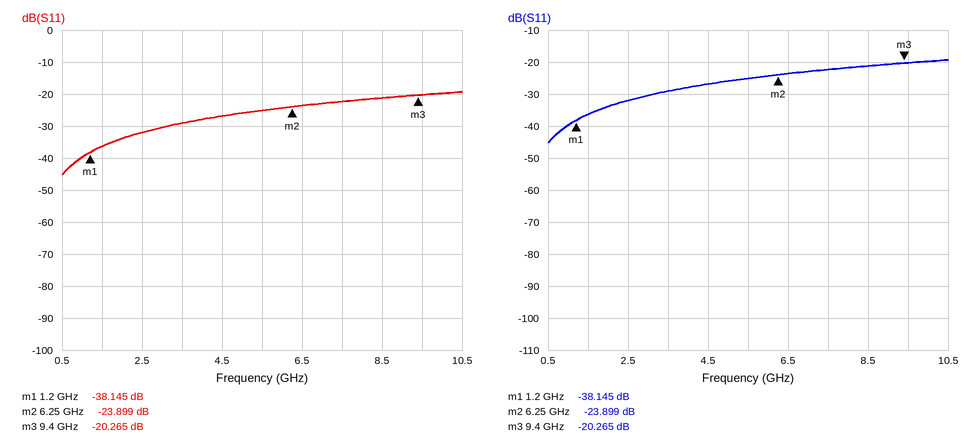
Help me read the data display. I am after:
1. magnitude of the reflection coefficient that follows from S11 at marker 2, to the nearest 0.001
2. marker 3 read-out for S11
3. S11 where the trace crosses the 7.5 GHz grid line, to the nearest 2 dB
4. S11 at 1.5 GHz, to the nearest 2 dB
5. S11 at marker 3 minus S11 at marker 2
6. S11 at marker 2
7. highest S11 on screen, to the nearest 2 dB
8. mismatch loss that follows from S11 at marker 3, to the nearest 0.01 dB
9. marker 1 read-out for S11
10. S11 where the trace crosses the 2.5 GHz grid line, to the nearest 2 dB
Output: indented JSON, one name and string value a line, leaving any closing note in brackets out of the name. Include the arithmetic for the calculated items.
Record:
{
  "magnitude of the reflection coefficient that follows from S11 at marker 2, to the nearest 0.001": "10^(-23.899/20) ≈ 0.064",
  "marker 3 read-out for S11": "-20.265 dB",
  "S11 where the trace crosses the 7.5 GHz grid line, to the nearest 2 dB": "-22 dB",
  "S11 at 1.5 GHz, to the nearest 2 dB": "-36 dB",
  "S11 at marker 3 minus S11 at marker 2": "-20.265 − (-23.899) = 3.634 dB",
  "S11 at marker 2": "-23.899 dB",
  "highest S11 on screen, to the nearest 2 dB": "-20 dB",
  "mismatch loss that follows from S11 at marker 3, to the nearest 0.01 dB": "−10 log10(1 − 10^(-20.265/10)) ≈ 0.04 dB",
  "marker 1 read-out for S11": "-38.145 dB",
  "S11 where the trace crosses the 2.5 GHz grid line, to the nearest 2 dB": "-32 dB"
}
